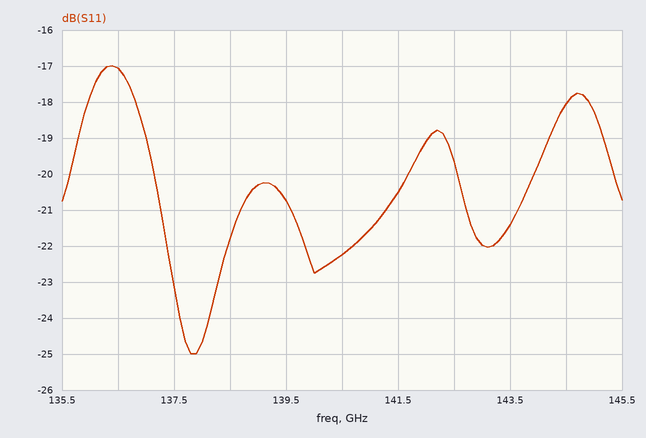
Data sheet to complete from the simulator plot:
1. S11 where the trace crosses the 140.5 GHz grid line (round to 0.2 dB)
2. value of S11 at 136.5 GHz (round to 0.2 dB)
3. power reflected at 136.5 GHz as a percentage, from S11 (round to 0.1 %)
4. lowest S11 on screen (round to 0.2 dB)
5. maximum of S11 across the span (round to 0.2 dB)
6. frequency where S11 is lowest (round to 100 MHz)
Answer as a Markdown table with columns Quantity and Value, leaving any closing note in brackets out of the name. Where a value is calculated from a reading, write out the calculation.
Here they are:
| Quantity | Value |
|---|---|
| S11 where the trace crosses the 140.5 GHz grid line | -22.2 dB |
| value of S11 at 136.5 GHz | -17.0 dB |
| power reflected at 136.5 GHz as a percentage, from S11 | 10^(-17/10) ≈ 2.0 % |
| lowest S11 on screen | -25.0 dB |
| maximum of S11 across the span | -17.0 dB |
| frequency where S11 is lowest | 137.8 GHz |
